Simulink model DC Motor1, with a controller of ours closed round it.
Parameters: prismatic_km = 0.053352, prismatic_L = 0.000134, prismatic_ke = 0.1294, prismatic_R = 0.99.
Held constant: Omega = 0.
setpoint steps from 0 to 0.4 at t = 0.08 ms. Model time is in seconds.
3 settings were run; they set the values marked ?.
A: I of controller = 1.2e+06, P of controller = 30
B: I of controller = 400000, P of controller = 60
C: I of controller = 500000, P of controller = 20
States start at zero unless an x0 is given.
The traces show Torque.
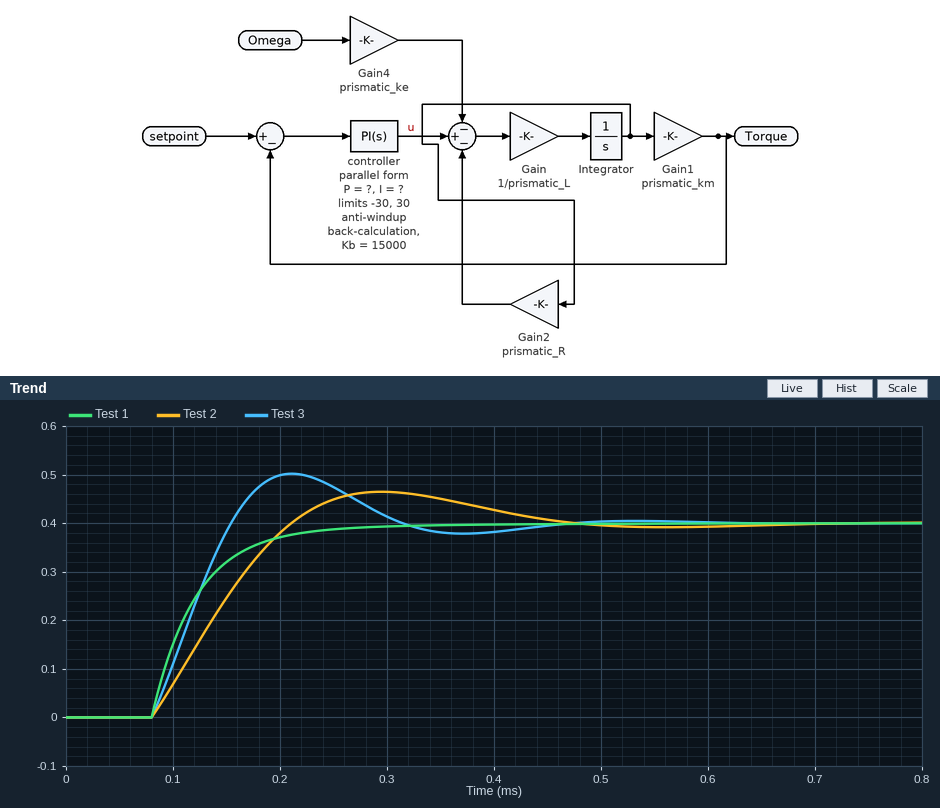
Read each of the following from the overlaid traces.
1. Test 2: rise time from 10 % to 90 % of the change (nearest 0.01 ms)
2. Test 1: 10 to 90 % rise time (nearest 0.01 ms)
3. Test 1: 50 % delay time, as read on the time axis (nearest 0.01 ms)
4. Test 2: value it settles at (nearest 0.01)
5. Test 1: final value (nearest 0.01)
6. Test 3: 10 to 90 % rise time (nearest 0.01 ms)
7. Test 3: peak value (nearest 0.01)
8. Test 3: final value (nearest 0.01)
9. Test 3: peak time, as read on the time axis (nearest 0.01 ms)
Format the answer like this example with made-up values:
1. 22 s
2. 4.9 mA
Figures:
1. 0.10 ms
2. 0.10 ms
3. 0.11 ms
4. 0.40
5. 0.40
6. 0.06 ms
7. 0.50
8. 0.40
9. 0.21 ms
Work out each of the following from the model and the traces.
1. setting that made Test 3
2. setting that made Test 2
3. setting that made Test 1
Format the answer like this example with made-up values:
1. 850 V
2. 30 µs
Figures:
1. A
2. C
3. B
